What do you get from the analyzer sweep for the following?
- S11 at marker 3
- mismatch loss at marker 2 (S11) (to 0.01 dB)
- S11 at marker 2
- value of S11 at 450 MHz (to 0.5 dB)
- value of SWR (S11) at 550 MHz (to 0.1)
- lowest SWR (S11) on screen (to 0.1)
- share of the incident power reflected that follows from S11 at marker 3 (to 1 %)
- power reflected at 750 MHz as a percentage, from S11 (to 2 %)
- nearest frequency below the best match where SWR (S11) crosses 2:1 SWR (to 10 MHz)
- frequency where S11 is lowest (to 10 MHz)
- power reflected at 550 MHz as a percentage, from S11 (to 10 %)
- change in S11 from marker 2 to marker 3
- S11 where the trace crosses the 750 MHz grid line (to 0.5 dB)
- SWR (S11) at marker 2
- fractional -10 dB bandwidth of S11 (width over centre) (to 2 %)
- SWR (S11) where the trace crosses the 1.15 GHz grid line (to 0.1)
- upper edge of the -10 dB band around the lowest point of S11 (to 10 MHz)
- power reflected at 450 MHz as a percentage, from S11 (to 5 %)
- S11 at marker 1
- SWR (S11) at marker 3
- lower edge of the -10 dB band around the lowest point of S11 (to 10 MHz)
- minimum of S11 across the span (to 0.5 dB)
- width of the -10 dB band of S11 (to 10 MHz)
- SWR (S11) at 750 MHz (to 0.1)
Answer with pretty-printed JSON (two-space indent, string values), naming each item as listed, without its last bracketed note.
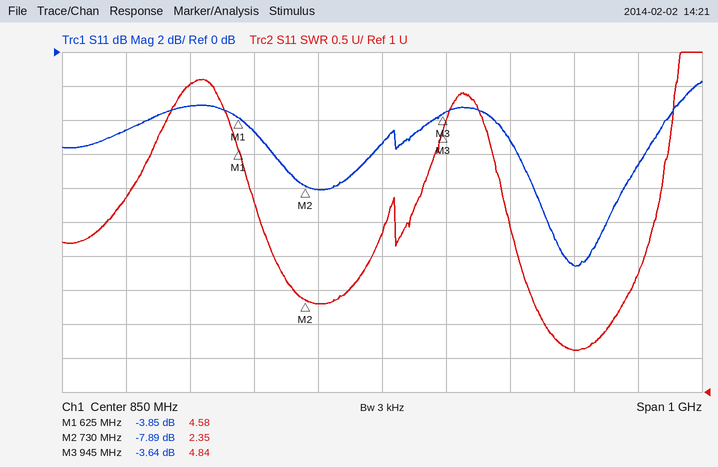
{
  "S11 at marker 3": "-3.64 dB",
  "mismatch loss at marker 2 (S11)": "0.77 dB",
  "S11 at marker 2": "-7.89 dB",
  "value of S11 at 450 MHz": "-4.5 dB",
  "value of SWR (S11) at 550 MHz": "5.5",
  "lowest SWR (S11) on screen": "1.6",
  "share of the incident power reflected that follows from S11 at marker 3": "43 %",
  "power reflected at 750 MHz as a percentage, from S11": "16 %",
  "nearest frequency below the best match where SWR (S11) crosses 2:1 SWR": "1.10 GHz",
  "frequency where S11 is lowest": "1.15 GHz",
  "power reflected at 550 MHz as a percentage, from S11": "50 %",
  "change in S11 from marker 2 to marker 3": "4.25 dB",
  "S11 where the trace crosses the 750 MHz grid line": "-8.0 dB",
  "SWR (S11) at marker 2": "2.35",
  "fractional -10 dB bandwidth of S11 (width over centre)": "8 %",
  "SWR (S11) where the trace crosses the 1.15 GHz grid line": "1.6",
  "upper edge of the -10 dB band around the lowest point of S11": "1.20 GHz",
  "power reflected at 450 MHz as a percentage, from S11": "35 %",
  "S11 at marker 1": "-3.85 dB",
  "SWR (S11) at marker 3": "4.84",
  "lower edge of the -10 dB band around the lowest point of S11": "1.11 GHz",
  "minimum of S11 across the span": "-12.5 dB",
  "width of the -10 dB band of S11": "90 MHz",
  "SWR (S11) at 750 MHz": "2.3"
}
